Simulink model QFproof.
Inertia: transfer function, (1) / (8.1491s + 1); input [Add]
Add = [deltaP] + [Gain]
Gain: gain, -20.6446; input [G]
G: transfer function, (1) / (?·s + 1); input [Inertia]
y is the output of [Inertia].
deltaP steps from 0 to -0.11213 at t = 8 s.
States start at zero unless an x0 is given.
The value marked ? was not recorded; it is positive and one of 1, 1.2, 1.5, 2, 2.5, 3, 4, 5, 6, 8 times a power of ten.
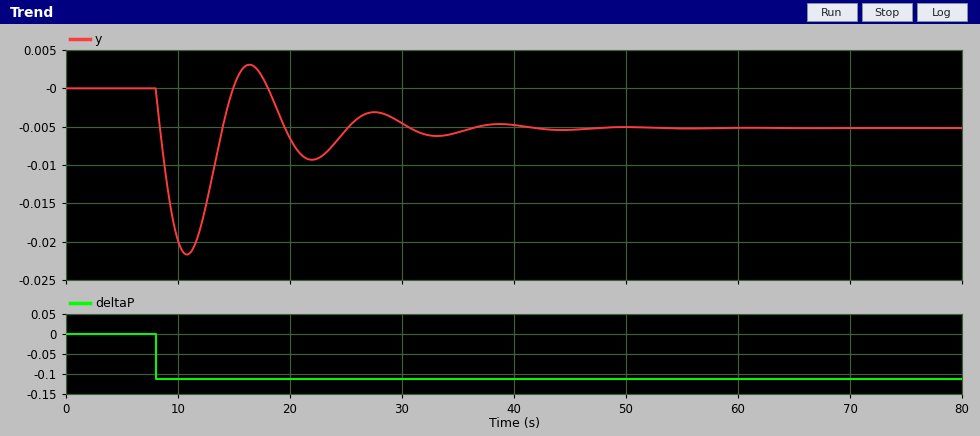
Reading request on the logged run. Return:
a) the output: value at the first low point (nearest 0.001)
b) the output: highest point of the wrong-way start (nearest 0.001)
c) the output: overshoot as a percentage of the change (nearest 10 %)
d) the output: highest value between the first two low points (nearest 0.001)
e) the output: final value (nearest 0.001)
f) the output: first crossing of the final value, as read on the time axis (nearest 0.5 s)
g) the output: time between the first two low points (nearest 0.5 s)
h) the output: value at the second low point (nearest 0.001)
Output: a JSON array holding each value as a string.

["-0.022", "0.003", "320 %", "0.003", "-0.005", "8.5 s", "11.0 s", "-0.009"]
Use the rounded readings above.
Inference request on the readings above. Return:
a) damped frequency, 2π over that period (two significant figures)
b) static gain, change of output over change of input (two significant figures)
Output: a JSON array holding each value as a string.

["0.57 rad/s", "0.045"]
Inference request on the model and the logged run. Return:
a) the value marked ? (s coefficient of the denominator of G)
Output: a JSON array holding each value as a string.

["8"]
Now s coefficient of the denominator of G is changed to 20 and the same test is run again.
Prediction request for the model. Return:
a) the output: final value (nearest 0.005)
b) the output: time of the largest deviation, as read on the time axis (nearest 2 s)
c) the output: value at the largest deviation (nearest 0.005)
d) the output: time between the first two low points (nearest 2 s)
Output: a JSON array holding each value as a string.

["-0.005", "12 s", "-0.030", "18 s"]
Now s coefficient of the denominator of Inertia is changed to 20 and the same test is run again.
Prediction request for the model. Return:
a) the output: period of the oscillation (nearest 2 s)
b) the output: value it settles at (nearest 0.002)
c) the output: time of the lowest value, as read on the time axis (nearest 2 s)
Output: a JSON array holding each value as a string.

["18 s", "-0.006", "12 s"]
